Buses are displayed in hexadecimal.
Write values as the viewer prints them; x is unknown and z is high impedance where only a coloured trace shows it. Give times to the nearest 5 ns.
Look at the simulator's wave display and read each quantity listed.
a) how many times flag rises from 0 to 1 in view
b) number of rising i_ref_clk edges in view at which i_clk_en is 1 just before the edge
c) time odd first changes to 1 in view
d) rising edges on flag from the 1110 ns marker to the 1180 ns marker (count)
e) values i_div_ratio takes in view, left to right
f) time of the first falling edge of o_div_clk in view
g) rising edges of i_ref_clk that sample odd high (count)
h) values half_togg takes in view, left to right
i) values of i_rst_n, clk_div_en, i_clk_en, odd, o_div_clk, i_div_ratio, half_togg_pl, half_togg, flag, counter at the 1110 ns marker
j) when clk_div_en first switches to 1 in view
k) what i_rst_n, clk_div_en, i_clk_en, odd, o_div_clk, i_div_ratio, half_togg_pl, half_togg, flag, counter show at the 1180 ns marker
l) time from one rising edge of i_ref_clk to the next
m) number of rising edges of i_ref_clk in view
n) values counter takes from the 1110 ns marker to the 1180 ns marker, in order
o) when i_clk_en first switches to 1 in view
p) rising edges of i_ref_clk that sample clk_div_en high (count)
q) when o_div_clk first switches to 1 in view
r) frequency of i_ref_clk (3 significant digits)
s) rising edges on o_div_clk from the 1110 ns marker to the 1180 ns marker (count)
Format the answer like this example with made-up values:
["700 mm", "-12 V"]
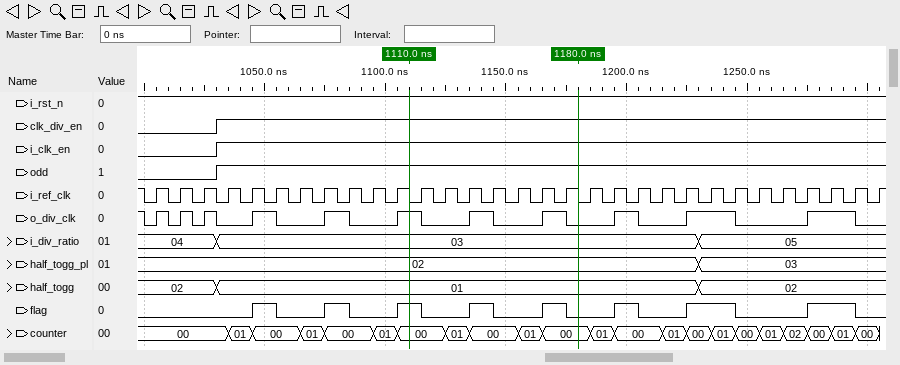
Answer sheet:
["8", "28", "1030 ns", "2", "04, 03, 05", "1000 ns", "28", "02, 01, 02", "i_rst_n=1, clk_div_en=1, i_clk_en=1, odd=1, o_div_clk=1, i_div_ratio=03, half_togg_pl=02, half_togg=01, flag=1, counter=00", "1030 ns", "i_rst_n=1, clk_div_en=1, i_clk_en=1, odd=1, o_div_clk=0, i_div_ratio=03, half_togg_pl=02, half_togg=01, flag=0, counter=00", "10 ns", "31", "00, 01, 00, 01, 00", "1030 ns", "28", "1005 ns", "100 MHz", "2"]
